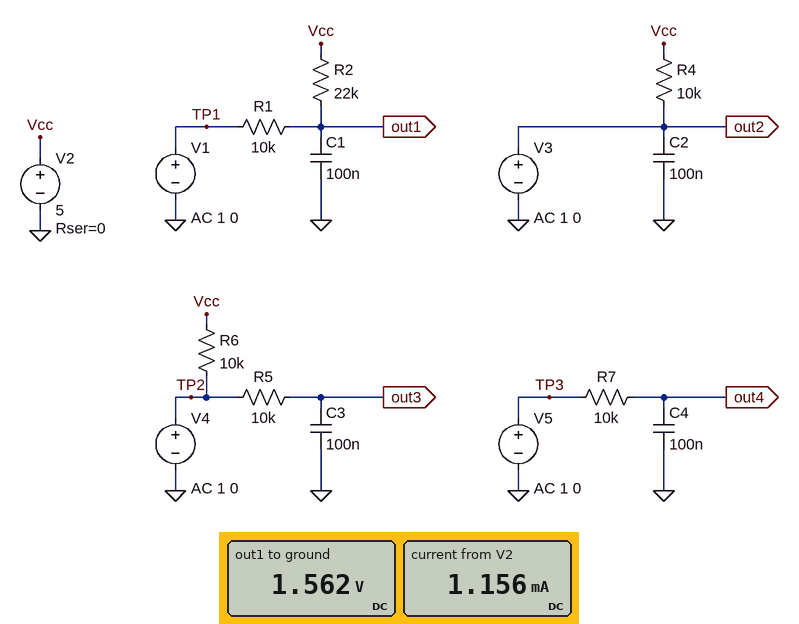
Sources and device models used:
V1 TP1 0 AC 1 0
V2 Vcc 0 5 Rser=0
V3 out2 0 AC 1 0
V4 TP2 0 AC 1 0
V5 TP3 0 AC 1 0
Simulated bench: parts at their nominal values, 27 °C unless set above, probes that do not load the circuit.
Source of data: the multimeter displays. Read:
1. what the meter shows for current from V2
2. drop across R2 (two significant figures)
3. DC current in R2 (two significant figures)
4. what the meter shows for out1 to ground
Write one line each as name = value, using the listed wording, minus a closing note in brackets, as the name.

what the meter shows for current from V2 = 1.156 mA
drop across R2 = 3.4 V
DC current in R2 = 160 µA
what the meter shows for out1 to ground = 1.562 V
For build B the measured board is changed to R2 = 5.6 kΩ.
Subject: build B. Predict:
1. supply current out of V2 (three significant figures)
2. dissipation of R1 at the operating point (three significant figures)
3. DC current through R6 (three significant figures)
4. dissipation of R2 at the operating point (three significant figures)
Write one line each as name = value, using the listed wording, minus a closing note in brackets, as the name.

supply current out of V2 = 1.32 mA
dissipation of R1 at the operating point = 1.03 mW
DC current through R6 = 500 µA
dissipation of R2 at the operating point = 575 µW
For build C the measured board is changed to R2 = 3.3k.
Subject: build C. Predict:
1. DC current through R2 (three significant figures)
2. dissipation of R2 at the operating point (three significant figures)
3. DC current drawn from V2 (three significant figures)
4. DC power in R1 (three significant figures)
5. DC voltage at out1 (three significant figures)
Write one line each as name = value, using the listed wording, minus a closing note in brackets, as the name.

DC current through R2 = 376 µA
dissipation of R2 at the operating point = 466 µW
DC current drawn from V2 = 1.38 mA
DC power in R1 = 1.41 mW
DC voltage at out1 = 3.76 V
